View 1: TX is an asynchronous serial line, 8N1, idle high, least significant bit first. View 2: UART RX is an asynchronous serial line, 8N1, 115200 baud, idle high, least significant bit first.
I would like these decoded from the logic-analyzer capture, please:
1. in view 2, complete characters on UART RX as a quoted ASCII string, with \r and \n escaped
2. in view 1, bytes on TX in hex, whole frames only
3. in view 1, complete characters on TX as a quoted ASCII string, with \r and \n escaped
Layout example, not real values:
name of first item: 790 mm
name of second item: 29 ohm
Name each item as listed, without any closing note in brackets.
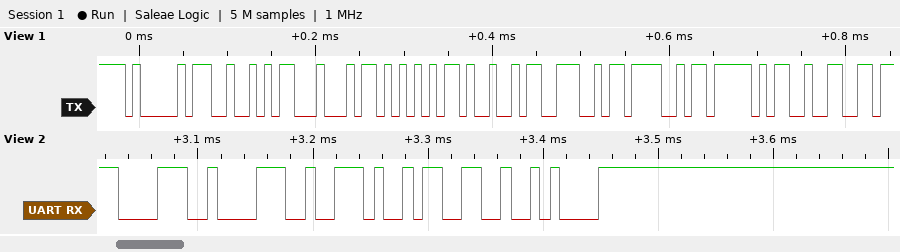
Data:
in view 2, complete characters on UART RX as a quoted ASCII string, with \r and \n escaped: "88.3\n"
in view 1, bytes on TX in hex, whole frames only: 0x41 0x52 0x44 0x55 0x49 0x4E 0x4F 0x5F 0x32
in view 1, complete characters on TX as a quoted ASCII string, with \r and \n escaped: "ARDUINO_2"
